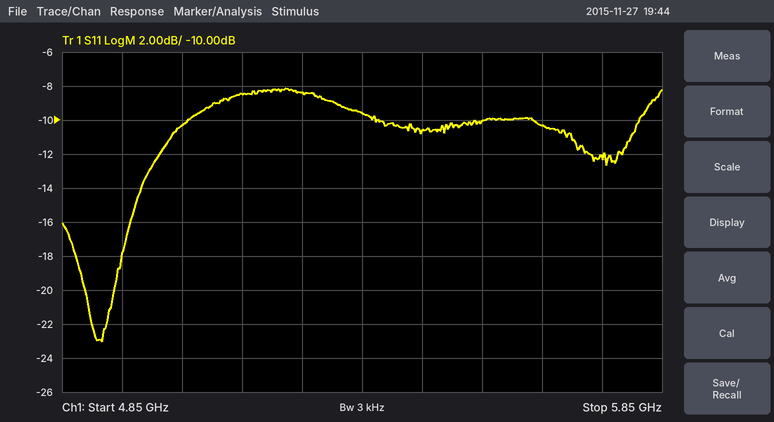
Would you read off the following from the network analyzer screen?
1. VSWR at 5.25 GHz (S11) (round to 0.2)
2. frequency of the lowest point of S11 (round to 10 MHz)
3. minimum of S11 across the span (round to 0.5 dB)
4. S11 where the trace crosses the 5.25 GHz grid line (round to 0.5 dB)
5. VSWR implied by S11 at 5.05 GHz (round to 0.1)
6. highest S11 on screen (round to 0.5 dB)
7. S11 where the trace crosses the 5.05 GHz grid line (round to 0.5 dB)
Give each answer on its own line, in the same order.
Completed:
2.2
4.92 GHz
-23.0 dB
-8.5 dB
1.9
-8.0 dB
-10.5 dB
